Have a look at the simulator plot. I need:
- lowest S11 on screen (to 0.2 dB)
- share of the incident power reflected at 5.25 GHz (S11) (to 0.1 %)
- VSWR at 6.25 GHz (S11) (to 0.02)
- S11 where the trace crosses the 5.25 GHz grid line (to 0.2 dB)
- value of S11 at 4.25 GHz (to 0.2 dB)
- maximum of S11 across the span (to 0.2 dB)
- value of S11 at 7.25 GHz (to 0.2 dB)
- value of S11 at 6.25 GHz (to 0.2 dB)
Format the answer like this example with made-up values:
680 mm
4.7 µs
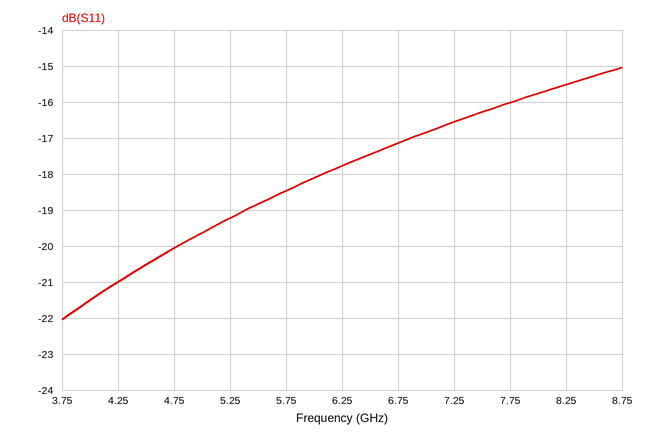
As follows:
-22.0 dB
1.2 %
1.30
-19.2 dB
-21.0 dB
-15.0 dB
-16.6 dB
-17.8 dB
